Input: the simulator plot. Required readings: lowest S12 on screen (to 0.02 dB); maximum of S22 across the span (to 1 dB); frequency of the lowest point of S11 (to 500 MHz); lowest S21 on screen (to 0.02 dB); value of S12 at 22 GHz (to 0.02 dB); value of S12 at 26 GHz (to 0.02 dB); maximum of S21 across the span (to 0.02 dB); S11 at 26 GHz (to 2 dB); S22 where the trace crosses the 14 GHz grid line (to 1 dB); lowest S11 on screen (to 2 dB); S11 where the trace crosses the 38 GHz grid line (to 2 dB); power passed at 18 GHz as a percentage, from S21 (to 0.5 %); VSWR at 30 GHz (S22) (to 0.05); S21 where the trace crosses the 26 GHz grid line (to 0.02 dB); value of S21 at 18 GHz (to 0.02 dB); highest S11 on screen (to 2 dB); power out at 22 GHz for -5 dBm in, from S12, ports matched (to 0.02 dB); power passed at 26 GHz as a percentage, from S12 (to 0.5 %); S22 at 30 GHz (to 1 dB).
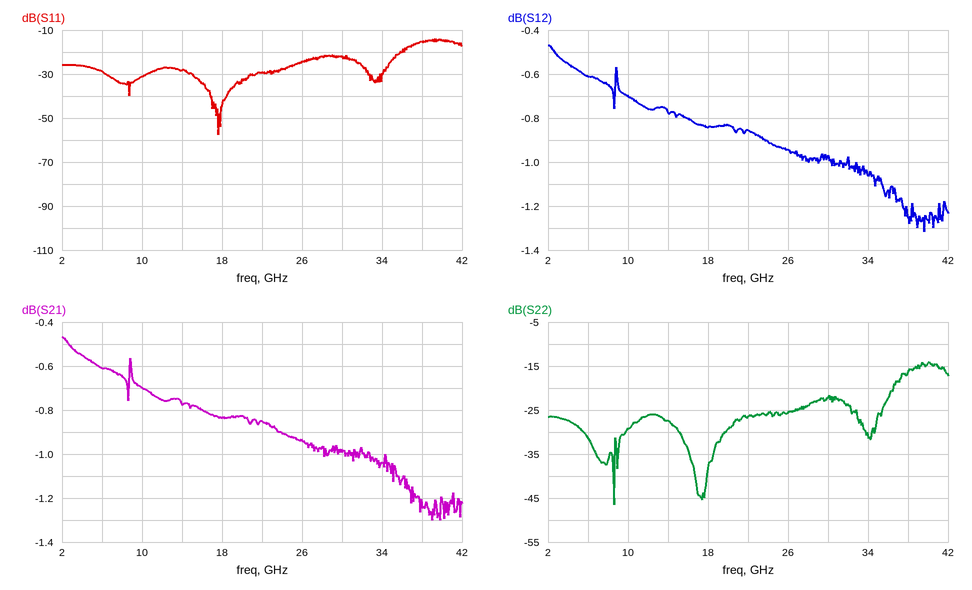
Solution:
-1.32 dB
-14 dB
17.5 GHz
-1.30 dB
-0.86 dB
-0.94 dB
-0.46 dB
-24 dB
-27 dB
-58 dB
-16 dB
82.5 %
1.15
-0.94 dB
-0.84 dB
-14 dB
-5.86 dBm
80.5 %
-22 dB
